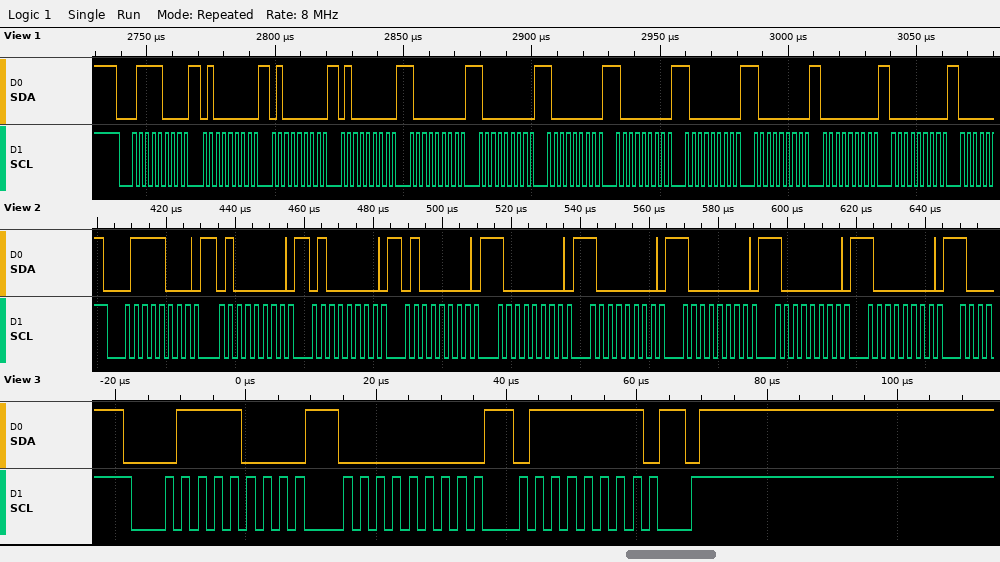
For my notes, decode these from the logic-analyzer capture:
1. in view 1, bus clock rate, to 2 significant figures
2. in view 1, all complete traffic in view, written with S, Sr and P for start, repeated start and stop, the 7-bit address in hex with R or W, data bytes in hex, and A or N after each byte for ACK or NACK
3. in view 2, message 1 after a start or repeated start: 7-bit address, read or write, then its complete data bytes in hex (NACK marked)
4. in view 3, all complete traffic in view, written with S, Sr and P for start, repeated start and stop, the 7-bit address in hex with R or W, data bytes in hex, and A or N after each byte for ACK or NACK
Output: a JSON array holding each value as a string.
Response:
["400 kHz", "S 3CW A 40 A 40 A 40 A 80 A 80 A 80 A 80 A 80 A 80 A 00 A 00 A", "0x3C write: 40 40 40 80 80 80 80 80", "S 3CW A 00 A 7F A P"]
